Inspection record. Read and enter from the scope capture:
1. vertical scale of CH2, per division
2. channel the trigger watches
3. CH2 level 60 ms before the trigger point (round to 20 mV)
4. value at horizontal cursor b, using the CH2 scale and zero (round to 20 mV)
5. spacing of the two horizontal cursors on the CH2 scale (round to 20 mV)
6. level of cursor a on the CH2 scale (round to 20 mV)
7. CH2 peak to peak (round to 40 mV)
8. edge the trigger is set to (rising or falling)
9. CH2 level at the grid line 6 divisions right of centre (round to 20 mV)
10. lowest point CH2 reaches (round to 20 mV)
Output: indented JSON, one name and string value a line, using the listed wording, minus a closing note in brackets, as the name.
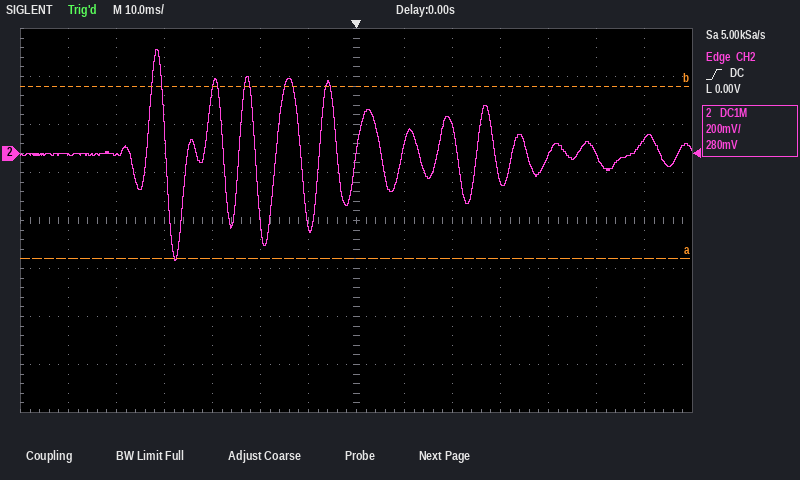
{
  "vertical scale of CH2, per division": "200 mV",
  "channel the trigger watches": "CH2",
  "CH2 level 60 ms before the trigger point": "0 mV",
  "value at horizontal cursor b, using the CH2 scale and zero": "280 mV",
  "spacing of the two horizontal cursors on the CH2 scale": "720 mV",
  "level of cursor a on the CH2 scale": "-440 mV",
  "CH2 peak to peak": "880 mV",
  "edge the trigger is set to": "rising",
  "CH2 level at the grid line 6 divisions right of centre": "60 mV",
  "lowest point CH2 reaches": "-440 mV"
}
